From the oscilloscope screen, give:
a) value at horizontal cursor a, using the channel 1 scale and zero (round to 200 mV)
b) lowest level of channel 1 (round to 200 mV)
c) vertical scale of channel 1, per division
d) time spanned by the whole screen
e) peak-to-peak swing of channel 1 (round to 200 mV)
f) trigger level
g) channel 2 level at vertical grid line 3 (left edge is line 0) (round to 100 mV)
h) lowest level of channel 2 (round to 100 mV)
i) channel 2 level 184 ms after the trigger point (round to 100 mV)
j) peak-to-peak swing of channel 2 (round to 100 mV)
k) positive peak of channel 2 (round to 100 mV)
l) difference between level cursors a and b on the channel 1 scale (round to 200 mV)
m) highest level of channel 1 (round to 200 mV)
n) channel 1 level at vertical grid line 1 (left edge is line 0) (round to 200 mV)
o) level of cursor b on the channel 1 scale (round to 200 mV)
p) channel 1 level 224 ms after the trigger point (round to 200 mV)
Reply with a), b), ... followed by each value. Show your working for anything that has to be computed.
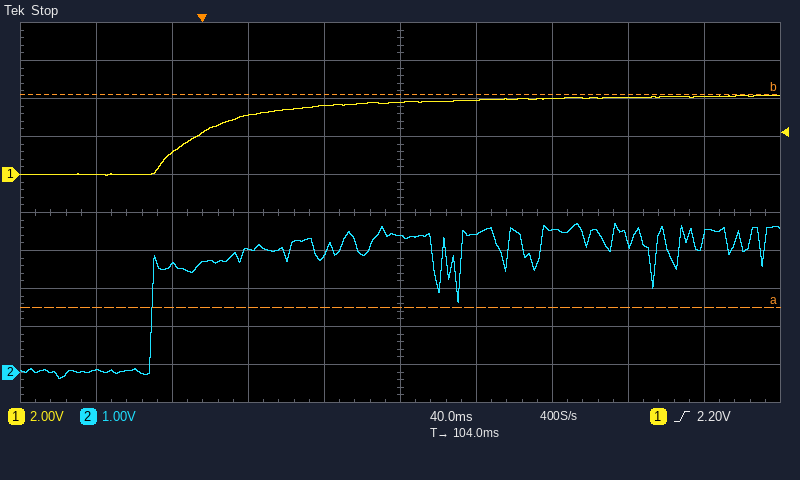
a) -7.0 V
b) 0.0 V
c) 2 V
d) 400 ms
e) 4.2 V − (0.0 V) = 4.2 V
f) 2.20 V
g) 3.2 V
h) -200 mV
i) 3.7 V
j) 3.9 V − (-200 mV) = 4.1 V
k) 3.9 V
l) 11.2 V
m) 4.2 V
n) 0.0 V
o) 4.2 V
p) 4.0 V
